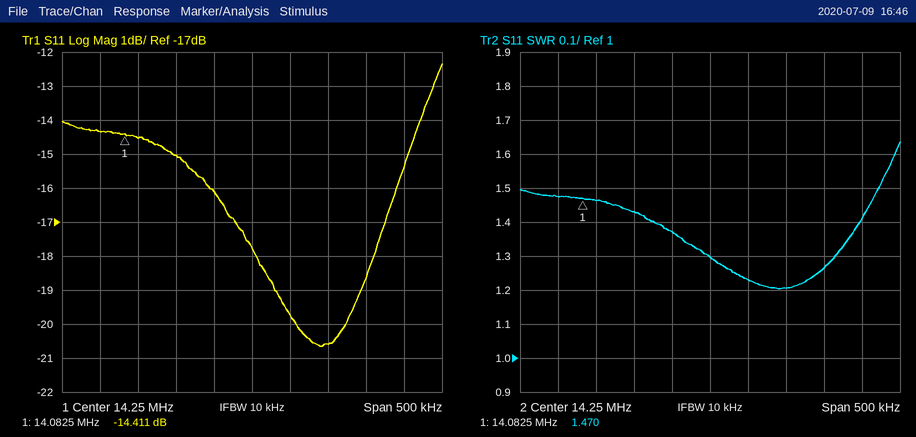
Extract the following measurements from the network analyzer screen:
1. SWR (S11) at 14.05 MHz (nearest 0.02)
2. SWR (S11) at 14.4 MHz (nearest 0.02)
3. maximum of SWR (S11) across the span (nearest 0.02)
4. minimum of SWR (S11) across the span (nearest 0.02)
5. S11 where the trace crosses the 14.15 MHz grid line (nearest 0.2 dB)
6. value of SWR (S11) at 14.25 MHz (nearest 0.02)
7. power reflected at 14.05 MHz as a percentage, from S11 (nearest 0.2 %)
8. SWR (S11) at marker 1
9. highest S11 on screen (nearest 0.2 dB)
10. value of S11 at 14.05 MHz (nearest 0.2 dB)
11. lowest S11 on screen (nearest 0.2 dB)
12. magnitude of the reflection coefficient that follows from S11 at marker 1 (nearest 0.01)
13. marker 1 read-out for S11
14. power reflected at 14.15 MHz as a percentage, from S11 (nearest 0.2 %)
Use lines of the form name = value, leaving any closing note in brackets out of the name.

SWR (S11) at 14.05 MHz = 1.48
SWR (S11) at 14.4 MHz = 1.26
maximum of SWR (S11) across the span = 1.64
minimum of SWR (S11) across the span = 1.20
S11 where the trace crosses the 14.15 MHz grid line = -15.0 dB
value of SWR (S11) at 14.25 MHz = 1.30
power reflected at 14.05 MHz as a percentage, from S11 = 3.6 %
SWR (S11) at marker 1 = 1.470
highest S11 on screen = -12.4 dB
value of S11 at 14.05 MHz = -14.4 dB
lowest S11 on screen = -20.6 dB
magnitude of the reflection coefficient that follows from S11 at marker 1 = 0.19
marker 1 read-out for S11 = -14.411 dB
power reflected at 14.15 MHz as a percentage, from S11 = 3.2 %
